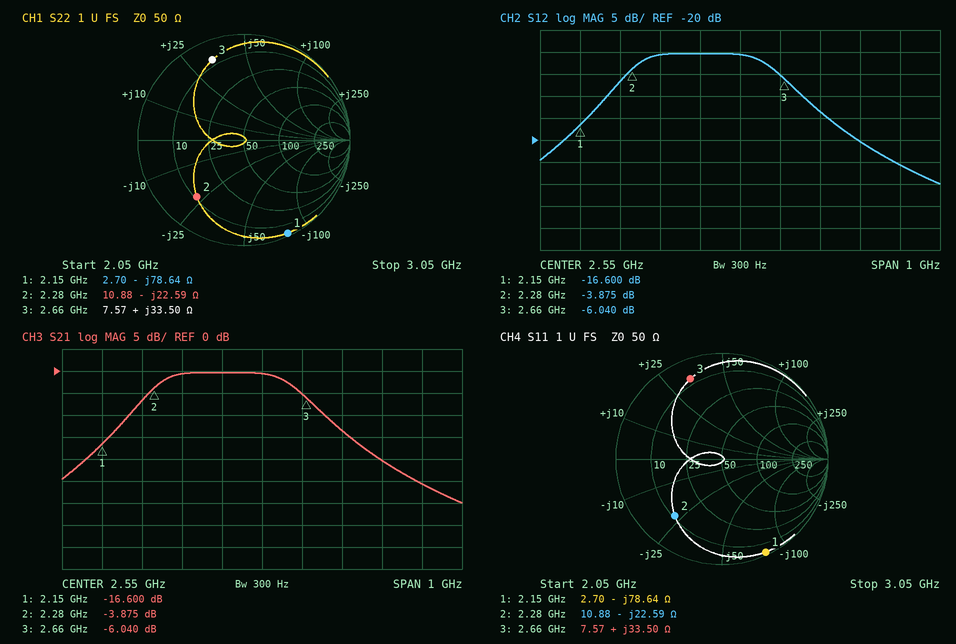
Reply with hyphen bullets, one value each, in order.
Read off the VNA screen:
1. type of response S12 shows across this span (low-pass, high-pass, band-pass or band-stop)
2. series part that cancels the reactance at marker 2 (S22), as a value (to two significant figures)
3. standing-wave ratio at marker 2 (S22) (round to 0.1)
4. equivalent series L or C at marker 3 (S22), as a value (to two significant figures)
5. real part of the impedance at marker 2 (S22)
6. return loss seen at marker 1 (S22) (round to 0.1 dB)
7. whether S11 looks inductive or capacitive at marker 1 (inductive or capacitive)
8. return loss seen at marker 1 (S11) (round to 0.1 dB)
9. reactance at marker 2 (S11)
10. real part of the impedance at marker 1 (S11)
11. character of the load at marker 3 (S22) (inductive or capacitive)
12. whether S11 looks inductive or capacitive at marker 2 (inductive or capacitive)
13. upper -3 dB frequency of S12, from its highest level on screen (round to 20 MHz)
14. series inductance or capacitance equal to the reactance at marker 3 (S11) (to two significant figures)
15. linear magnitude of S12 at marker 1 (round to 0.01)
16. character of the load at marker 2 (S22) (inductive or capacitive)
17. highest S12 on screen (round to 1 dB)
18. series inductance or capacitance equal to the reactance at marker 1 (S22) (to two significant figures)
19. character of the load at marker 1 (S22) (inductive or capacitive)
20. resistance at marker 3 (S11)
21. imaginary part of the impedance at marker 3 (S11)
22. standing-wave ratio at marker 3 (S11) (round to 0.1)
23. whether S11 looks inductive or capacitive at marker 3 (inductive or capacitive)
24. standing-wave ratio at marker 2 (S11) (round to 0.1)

- band-pass
- 1.6 nH
- 5.6
- 2.0 nH
- 10.88 Ω
- 0.3 dB
- capacitive
- 0.3 dB
- -22.59 Ω
- 2.70 Ω
- inductive
- capacitive
- 2.62 GHz
- 2.0 nH
- 0.15
- capacitive
- 0 dB
- 940 fF
- capacitive
- 7.57 Ω
- +33.50 Ω
- 9.6
- inductive
- 5.6
